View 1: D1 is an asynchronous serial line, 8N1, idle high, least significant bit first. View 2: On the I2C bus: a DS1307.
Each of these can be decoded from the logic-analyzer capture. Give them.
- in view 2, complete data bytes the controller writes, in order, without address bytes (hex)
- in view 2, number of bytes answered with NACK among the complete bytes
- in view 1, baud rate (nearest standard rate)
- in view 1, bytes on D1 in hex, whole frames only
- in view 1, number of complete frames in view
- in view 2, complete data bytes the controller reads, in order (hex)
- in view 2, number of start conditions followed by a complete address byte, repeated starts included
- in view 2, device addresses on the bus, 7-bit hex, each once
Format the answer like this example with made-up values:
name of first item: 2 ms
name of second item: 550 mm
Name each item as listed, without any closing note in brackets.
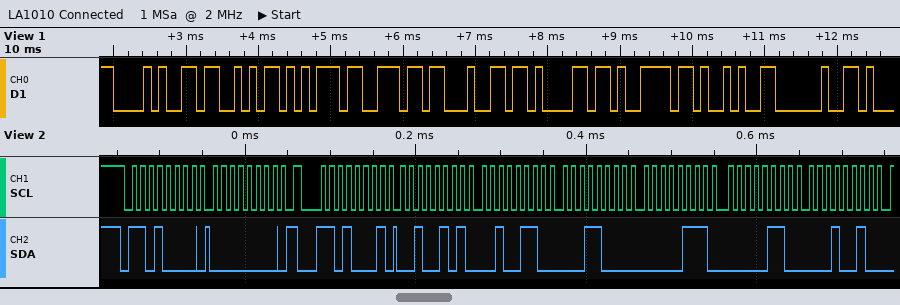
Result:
in view 2, complete data bytes the controller writes, in order, without address bytes: 00
in view 2, number of bytes answered with NACK among the complete bytes: 0
in view 1, baud rate: 9600 baud
in view 1, bytes on D1 in hex, whole frames only: 28 53 75 6E 64 61 79 29 20
in view 1, number of complete frames in view: 9
in view 2, complete data bytes the controller reads, in order: 25 26 18 07 06 12
in view 2, number of start conditions followed by a complete address byte, repeated starts included: 2
in view 2, device addresses on the bus, 7-bit hex, each once: 0x68
